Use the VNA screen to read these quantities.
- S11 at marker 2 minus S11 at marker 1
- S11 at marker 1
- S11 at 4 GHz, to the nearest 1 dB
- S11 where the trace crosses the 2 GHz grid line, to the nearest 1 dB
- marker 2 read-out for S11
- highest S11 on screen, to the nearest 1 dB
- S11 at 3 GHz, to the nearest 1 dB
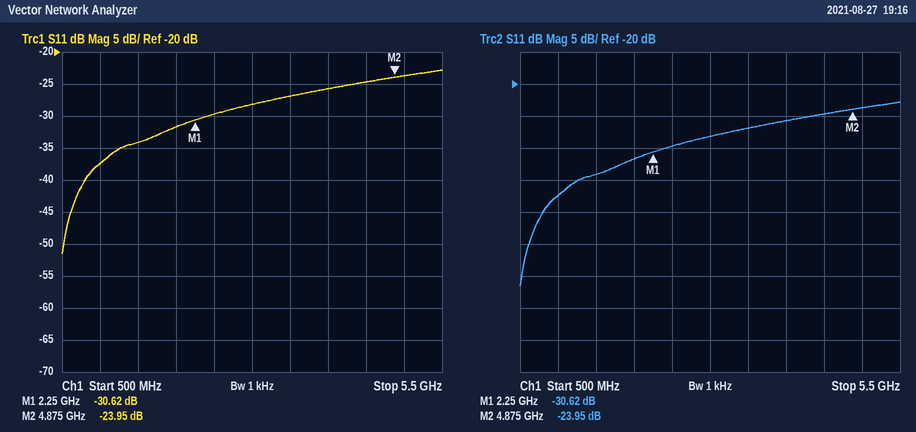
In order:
6.67 dB
-30.62 dB
-26 dB
-32 dB
-23.95 dB
-23 dB
-28 dB
